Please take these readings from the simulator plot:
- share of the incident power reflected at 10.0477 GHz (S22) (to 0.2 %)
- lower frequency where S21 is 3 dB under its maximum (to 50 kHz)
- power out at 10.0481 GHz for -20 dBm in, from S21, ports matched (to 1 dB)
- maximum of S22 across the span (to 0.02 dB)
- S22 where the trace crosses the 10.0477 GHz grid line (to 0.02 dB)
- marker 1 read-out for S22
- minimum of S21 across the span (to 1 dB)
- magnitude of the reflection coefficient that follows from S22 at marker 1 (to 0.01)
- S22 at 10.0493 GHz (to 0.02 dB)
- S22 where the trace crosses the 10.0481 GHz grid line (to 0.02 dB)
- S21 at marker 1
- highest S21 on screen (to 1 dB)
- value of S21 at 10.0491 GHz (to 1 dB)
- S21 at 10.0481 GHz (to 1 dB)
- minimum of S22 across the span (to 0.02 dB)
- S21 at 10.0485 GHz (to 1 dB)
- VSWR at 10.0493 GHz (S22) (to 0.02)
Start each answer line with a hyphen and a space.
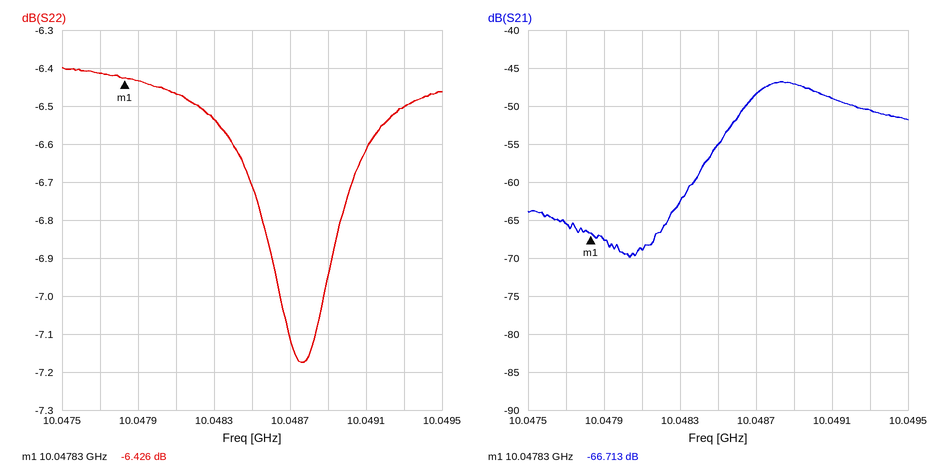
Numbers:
- 22.8 %
- 10.04865 GHz
- -89 dBm
- -6.40 dB
- -6.42 dB
- -6.426 dB
- -70 dB
- 0.48
- -6.50 dB
- -6.46 dB
- -66.713 dB
- -47 dB
- -49 dB
- -69 dB
- -7.18 dB
- -55 dB
- 2.80
